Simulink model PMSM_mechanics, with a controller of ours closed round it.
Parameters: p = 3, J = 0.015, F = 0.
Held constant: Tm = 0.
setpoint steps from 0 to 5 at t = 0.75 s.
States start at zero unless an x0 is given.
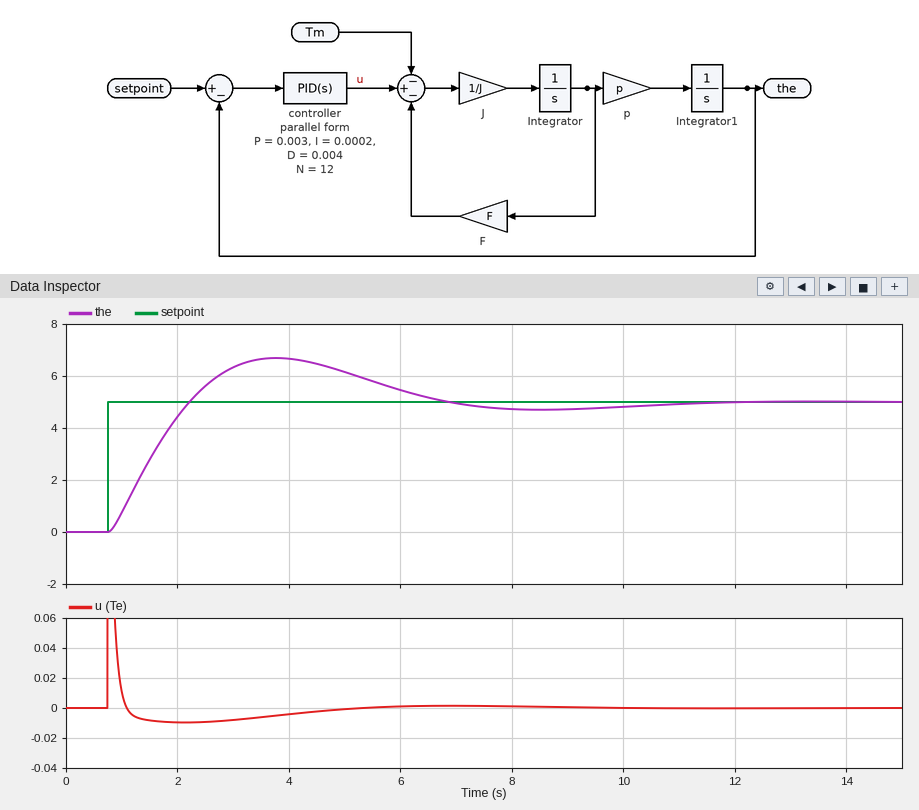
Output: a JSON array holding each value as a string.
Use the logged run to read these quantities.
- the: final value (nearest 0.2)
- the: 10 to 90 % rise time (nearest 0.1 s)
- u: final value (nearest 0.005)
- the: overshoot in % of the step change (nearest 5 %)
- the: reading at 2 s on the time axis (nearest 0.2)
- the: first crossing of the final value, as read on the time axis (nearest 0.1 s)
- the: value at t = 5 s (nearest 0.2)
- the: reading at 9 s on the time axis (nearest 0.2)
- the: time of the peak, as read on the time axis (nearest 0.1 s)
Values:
["5.0", "1.1 s", "0.000", "35 %", "4.4", "2.2 s", "6.2", "4.8", "3.8 s"]
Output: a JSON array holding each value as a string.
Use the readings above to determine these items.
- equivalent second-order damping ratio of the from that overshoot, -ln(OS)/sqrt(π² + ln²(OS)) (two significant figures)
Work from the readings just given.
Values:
["0.32"]
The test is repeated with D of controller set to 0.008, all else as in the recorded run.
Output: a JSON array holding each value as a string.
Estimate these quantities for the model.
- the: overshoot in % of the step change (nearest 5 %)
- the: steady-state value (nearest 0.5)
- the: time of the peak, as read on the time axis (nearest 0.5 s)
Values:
["15 %", "5.0", "3.0 s"]
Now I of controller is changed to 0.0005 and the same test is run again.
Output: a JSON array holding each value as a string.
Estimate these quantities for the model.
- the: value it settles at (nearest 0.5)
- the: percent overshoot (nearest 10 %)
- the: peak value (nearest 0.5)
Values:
["5.0", "40 %", "7.0"]
